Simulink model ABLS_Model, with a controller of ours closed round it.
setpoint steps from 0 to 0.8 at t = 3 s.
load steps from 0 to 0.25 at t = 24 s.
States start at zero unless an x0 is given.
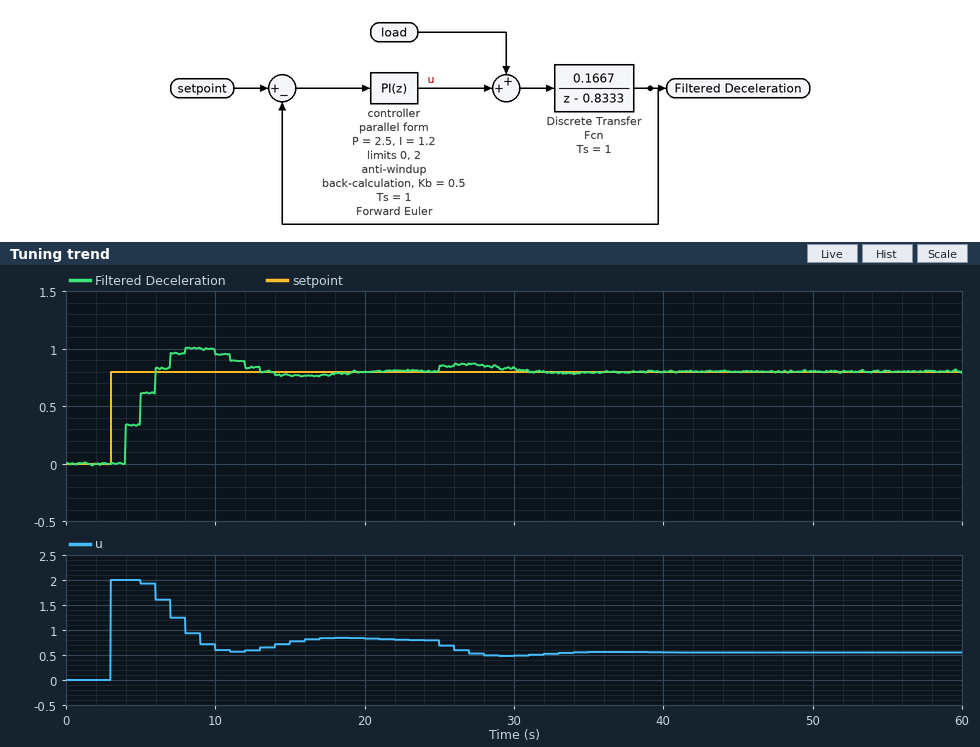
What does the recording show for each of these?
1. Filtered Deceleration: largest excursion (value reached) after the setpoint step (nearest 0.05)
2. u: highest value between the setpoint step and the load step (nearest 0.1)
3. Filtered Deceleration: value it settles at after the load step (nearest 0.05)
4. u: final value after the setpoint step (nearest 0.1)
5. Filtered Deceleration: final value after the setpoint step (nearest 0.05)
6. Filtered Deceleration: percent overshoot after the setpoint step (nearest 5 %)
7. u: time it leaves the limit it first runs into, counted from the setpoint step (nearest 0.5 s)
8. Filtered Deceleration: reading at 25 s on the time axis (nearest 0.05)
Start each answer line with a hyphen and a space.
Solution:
- 1.00
- 2.0
- 0.80
- 0.8
- 0.80
- 25 %
- 2.0 s
- 0.85
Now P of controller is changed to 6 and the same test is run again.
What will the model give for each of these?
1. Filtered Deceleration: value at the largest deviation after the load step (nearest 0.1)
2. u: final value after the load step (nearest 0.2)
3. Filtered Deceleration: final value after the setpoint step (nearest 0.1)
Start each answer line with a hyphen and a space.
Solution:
- 0.8
- 0.6
- 0.8
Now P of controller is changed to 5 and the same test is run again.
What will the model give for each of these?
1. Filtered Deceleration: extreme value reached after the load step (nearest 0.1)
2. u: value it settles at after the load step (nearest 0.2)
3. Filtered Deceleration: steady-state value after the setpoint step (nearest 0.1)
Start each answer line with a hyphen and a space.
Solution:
- 0.8
- 0.6
- 0.8
